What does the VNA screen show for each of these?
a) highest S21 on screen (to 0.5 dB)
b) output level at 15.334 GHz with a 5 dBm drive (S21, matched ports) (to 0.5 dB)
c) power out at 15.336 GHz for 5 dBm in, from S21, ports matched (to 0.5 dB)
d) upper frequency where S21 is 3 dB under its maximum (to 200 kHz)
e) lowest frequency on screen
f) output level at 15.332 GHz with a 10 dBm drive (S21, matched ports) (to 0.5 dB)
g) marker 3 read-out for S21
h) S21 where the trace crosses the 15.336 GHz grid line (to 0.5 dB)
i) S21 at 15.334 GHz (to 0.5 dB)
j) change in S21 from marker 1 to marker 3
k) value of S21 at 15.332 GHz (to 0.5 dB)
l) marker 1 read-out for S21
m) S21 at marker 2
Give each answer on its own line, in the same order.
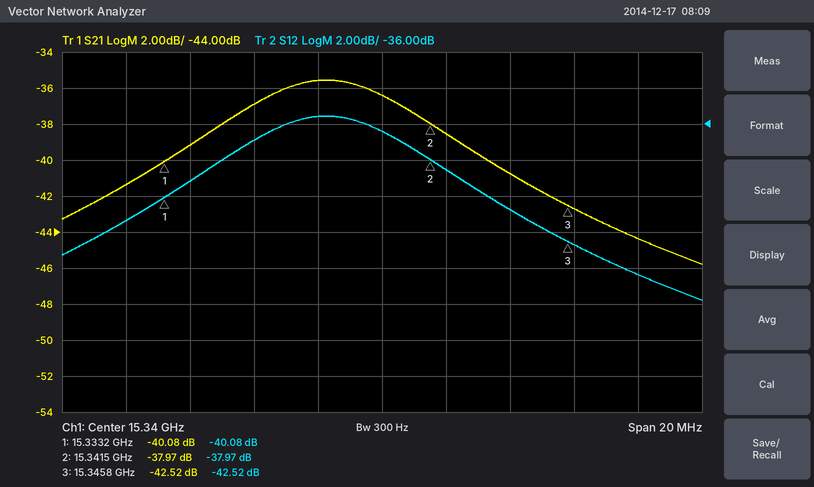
-35.5 dB
-34.0 dBm
-32.0 dBm
15.3420 GHz
15.33 GHz
-31.5 dBm
-42.52 dB
-37.0 dB
-39.0 dB
-2.44 dB
-41.5 dB
-40.08 dB
-37.97 dB
